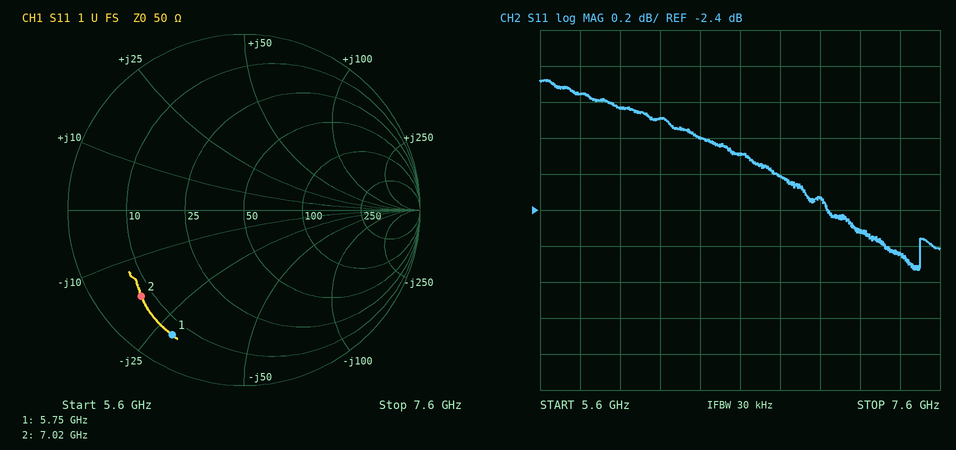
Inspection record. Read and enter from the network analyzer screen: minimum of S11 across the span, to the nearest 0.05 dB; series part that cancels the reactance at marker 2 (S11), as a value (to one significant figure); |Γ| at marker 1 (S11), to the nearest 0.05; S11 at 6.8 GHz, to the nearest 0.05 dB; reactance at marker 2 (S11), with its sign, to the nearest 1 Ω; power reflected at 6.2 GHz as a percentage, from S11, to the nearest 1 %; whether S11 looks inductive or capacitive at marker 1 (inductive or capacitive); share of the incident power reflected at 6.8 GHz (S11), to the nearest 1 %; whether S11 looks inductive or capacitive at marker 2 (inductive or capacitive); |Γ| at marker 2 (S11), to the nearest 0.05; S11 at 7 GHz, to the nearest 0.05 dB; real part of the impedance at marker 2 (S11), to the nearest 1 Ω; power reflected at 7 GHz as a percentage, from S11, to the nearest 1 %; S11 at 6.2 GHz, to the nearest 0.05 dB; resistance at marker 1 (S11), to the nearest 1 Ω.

-2.75 dB
400 pH
0.80
-2.20 dB
-18 Ω
65 %
capacitive
60 %
capacitive
0.75
-2.35 dB
8 Ω
58 %
-1.90 dB
7 Ω
